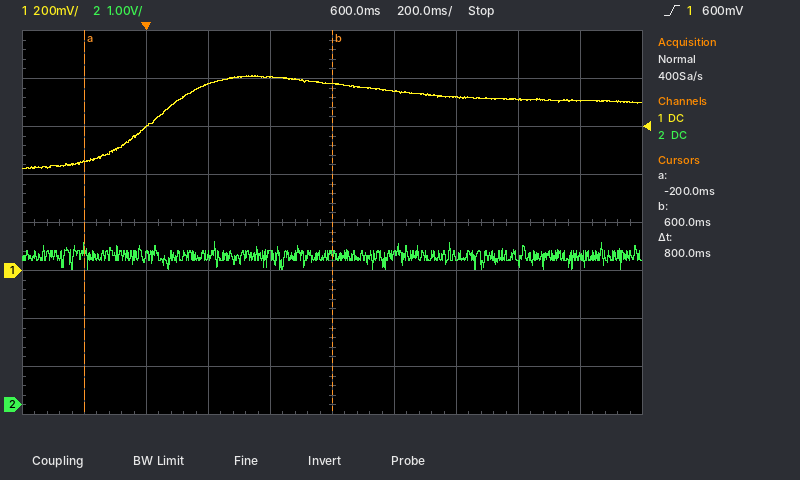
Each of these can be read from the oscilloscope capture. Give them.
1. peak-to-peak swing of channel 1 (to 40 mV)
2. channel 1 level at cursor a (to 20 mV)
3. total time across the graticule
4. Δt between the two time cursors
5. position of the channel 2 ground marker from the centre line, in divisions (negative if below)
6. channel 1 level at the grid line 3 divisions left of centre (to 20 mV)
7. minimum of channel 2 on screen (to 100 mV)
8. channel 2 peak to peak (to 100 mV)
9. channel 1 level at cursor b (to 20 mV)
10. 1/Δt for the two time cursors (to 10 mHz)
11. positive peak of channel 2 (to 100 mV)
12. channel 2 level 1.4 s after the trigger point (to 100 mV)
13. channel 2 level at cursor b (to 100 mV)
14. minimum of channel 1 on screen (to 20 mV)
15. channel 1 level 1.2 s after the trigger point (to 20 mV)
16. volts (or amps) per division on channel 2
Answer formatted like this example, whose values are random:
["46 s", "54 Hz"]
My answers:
["400 mV", "460 mV", "2 s", "800 ms", "-3.8 div", "600 mV", "2.8 V", "600 mV", "780 mV", "1.25 Hz", "3.4 V", "3.1 V", "3.1 V", "420 mV", "720 mV", "1 V"]
